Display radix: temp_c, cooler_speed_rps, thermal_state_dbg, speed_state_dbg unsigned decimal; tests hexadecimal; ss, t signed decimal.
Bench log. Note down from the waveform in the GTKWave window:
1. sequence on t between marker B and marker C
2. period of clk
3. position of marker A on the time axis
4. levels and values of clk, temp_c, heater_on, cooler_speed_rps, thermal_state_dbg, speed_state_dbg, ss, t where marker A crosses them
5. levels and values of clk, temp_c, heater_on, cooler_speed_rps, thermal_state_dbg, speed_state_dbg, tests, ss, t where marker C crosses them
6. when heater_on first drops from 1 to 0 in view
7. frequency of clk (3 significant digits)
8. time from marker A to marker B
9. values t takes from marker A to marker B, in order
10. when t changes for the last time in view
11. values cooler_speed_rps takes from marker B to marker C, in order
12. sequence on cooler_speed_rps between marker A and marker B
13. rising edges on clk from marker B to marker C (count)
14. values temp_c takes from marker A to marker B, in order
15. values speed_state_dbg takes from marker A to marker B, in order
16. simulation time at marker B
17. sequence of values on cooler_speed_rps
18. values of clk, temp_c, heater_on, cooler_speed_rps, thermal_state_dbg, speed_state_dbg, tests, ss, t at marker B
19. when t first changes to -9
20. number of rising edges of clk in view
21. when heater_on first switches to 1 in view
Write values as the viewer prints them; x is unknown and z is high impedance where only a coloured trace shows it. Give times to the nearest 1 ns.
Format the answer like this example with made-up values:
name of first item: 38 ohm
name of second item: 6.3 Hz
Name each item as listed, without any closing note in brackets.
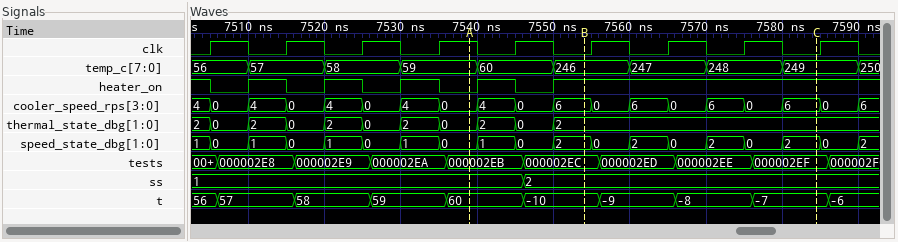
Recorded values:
sequence on t between marker B and marker C: -10, -9, -8, -7
period of clk: 10 ns
position of marker A on the time axis: 7539 ns
levels and values of clk, temp_c, heater_on, cooler_speed_rps, thermal_state_dbg, speed_state_dbg, ss, t where marker A crosses them: clk=1, temp_c=59, heater_on=0, cooler_speed_rps=0, thermal_state_dbg=0, speed_state_dbg=0, ss=1, t=60
levels and values of clk, temp_c, heater_on, cooler_speed_rps, thermal_state_dbg, speed_state_dbg, tests, ss, t where marker C crosses them: clk=0, temp_c=249, heater_on=1, cooler_speed_rps=6, thermal_state_dbg=2, speed_state_dbg=2, tests=000002EF, ss=2, t=-7
when heater_on first drops from 1 to 0 in view: 7505 ns
frequency of clk: 100 MHz
time from marker A to marker B: 15 ns
values t takes from marker A to marker B, in order: 60, -10
when t changes for the last time in view: 7586 ns
values cooler_speed_rps takes from marker B to marker C, in order: 6, 0, 6, 0, 6, 0, 6
sequence on cooler_speed_rps between marker A and marker B: 0, 4, 0, 6
rising edges on clk from marker B to marker C: 3
values temp_c takes from marker A to marker B, in order: 59, 60, 246
values speed_state_dbg takes from marker A to marker B, in order: 0, 1, 0, 2
simulation time at marker B: 7554 ns
sequence of values on cooler_speed_rps: 4, 0, 4, 0, 4, 0, 4, 0, 4, 0, 6, 0, 6, 0, 6, 0, 6, 0, 6
values of clk, temp_c, heater_on, cooler_speed_rps, thermal_state_dbg, speed_state_dbg, tests, ss, t at marker B: clk=0, temp_c=246, heater_on=1, cooler_speed_rps=6, thermal_state_dbg=2, speed_state_dbg=2, tests=000002EC, ss=2, t=-10
when t first changes to -9: 7556 ns
number of rising edges of clk in view: 9
when heater_on first switches to 1 in view: 7510 ns
